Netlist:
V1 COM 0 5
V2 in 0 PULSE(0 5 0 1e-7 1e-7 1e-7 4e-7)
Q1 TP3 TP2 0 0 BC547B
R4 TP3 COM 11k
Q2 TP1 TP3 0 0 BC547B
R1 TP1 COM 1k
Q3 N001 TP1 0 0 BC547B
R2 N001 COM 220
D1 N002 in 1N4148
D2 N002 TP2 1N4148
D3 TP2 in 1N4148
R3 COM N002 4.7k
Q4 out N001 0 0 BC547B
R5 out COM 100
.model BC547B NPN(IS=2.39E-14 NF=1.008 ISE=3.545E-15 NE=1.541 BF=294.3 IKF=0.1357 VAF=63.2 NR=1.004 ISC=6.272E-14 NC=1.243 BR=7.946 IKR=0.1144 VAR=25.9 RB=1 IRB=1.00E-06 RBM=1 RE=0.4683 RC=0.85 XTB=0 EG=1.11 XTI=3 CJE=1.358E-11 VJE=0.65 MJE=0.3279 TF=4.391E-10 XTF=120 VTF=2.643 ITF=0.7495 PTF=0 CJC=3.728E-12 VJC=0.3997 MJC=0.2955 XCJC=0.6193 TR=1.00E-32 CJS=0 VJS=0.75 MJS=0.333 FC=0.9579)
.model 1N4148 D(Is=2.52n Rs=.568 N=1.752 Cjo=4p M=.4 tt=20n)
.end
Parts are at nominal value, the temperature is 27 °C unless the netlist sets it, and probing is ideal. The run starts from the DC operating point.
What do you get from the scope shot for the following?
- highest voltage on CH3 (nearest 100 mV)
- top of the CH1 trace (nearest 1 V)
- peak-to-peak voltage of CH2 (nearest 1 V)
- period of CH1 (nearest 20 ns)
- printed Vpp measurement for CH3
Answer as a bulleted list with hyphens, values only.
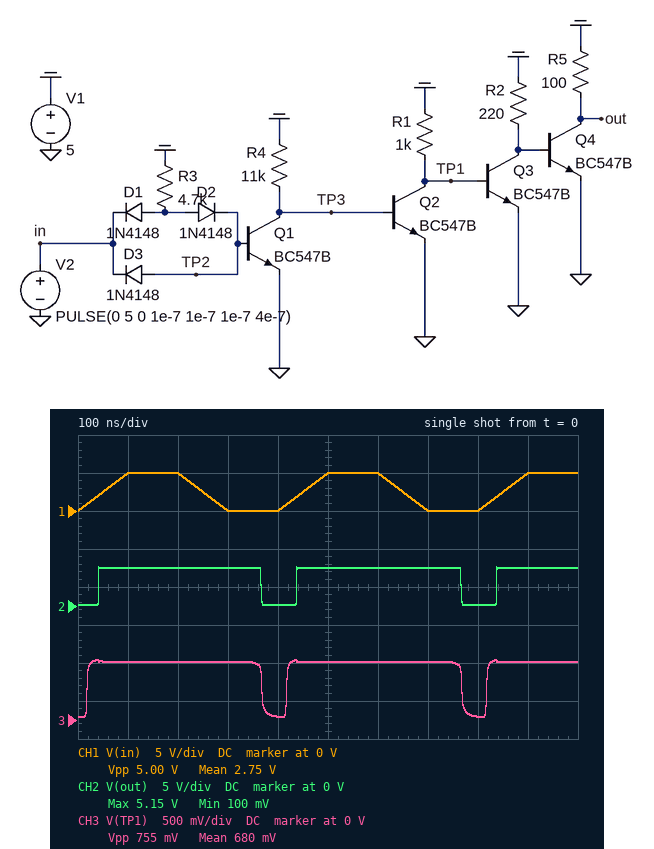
- 800 mV
- 5 V
- 5 V
- 400 ns
- 755 mV
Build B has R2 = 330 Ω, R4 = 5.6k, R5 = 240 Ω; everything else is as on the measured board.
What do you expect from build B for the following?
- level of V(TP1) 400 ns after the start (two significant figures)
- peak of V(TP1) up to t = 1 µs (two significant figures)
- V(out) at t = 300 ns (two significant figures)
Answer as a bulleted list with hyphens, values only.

- 31 mV
- 770 mV
- 5.0 V
